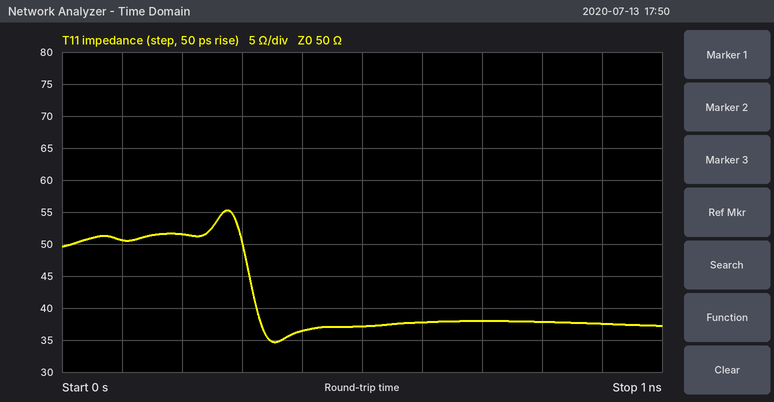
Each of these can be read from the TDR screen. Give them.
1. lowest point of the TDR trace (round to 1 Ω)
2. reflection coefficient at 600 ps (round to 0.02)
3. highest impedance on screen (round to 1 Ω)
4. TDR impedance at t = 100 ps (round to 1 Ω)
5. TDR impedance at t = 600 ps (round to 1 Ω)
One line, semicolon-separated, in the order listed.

35 Ω; -0.14; 55 Ω; 51 Ω; 38 Ω
